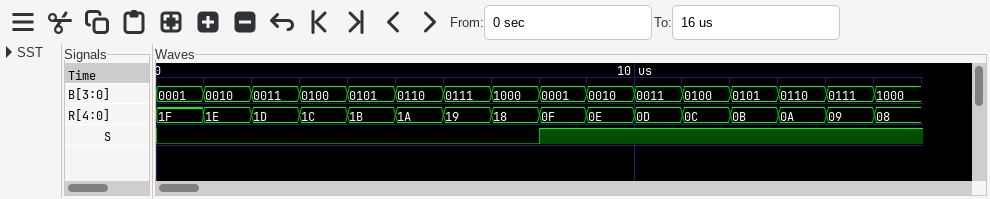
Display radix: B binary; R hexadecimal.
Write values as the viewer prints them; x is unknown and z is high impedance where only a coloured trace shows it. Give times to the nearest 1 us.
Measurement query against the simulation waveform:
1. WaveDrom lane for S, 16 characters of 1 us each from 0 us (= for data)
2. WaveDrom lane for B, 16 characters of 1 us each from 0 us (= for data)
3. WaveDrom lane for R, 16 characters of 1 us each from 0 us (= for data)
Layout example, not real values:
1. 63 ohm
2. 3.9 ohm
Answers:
1. {name: 'S', wave: '0.......1.......'}
2. {name: 'B', wave: '================', data: '0001 0010 0011 0100 0101 0110 0111 1000 0001 0010 0011 0100 0101 0110 0111 1000'}
3. {name: 'R', wave: '================', data: '1F 1E 1D 1C 1B 1A 19 18 0F 0E 0D 0C 0B 0A 09 08'}
